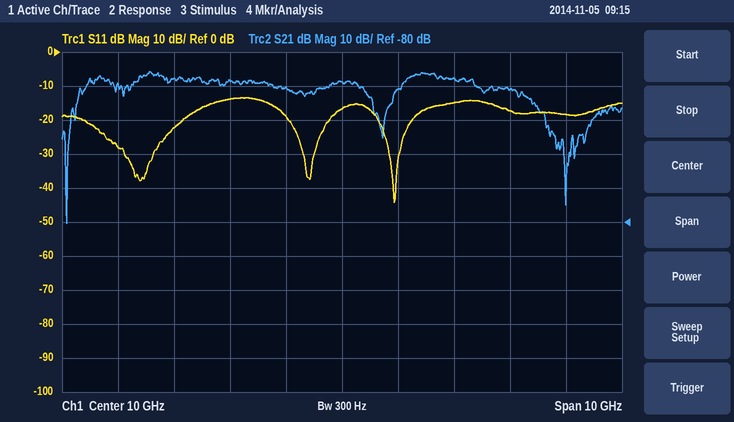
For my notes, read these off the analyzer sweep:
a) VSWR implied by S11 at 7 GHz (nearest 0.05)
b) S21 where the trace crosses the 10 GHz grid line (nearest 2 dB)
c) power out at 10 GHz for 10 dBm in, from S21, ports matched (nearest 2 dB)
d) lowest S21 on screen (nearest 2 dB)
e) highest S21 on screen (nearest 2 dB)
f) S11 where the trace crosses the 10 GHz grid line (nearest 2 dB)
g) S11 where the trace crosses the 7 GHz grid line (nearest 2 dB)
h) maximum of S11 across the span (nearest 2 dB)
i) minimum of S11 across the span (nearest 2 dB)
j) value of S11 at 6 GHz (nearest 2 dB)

1.15
-38 dB
-28 dBm
-80 dB
-36 dB
-16 dB
-22 dB
-14 dB
-44 dB
-28 dB
